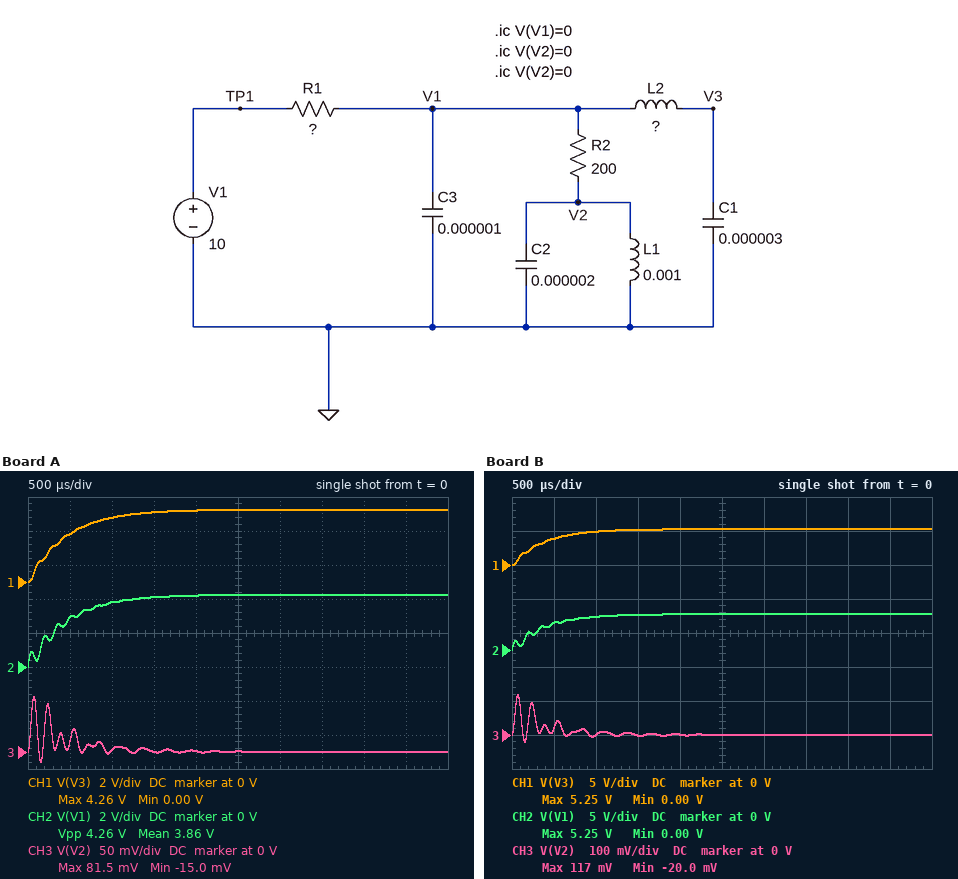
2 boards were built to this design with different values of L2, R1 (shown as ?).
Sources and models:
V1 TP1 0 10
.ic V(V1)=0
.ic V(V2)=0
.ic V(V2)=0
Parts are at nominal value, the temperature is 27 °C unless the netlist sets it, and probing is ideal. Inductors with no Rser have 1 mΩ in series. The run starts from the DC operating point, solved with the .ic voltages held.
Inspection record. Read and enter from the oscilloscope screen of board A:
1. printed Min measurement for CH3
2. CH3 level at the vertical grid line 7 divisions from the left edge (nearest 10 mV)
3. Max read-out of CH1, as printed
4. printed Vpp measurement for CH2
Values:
-15.0 mV
0 V
4.26 V
4.26 V
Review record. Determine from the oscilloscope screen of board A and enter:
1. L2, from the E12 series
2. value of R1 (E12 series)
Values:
820 µH
270 Ω
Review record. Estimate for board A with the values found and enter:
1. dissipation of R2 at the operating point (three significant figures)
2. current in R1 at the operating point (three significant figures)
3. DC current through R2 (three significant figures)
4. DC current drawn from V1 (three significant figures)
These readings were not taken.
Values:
90.5 mW
21.3 mA
21.3 mA
21.3 mA
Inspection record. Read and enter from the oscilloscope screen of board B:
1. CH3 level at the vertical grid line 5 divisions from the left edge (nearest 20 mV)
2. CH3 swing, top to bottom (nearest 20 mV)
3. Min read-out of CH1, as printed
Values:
0 V
140 mV
0.00 V
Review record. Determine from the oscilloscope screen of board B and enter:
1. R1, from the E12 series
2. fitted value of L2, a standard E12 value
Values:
180 Ω
820 µH
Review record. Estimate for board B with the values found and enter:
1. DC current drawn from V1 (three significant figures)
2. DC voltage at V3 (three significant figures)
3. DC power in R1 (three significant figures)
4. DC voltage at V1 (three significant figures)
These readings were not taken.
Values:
26.3 mA
5.26 V
125 mW
5.26 V
